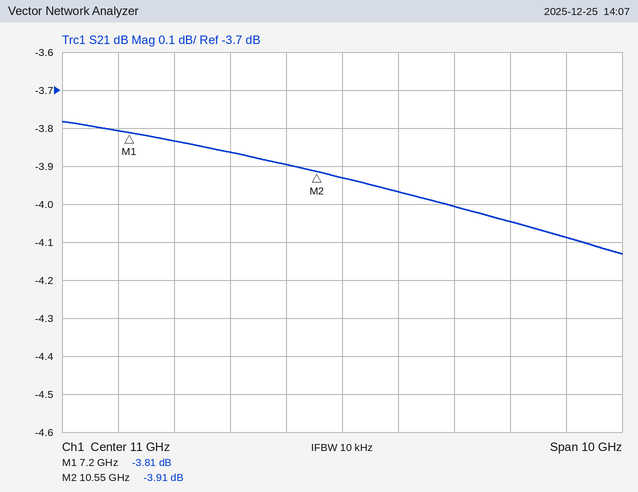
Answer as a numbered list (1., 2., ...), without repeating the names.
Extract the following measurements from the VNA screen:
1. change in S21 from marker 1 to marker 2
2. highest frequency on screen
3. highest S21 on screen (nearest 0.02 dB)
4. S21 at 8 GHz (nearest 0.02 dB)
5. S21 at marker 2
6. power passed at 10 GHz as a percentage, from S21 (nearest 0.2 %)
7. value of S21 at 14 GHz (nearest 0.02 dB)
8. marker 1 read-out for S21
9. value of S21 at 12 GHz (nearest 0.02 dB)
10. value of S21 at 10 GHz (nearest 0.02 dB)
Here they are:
1. -0.10 dB
2. 16 GHz
3. -3.78 dB
4. -3.84 dB
5. -3.91 dB
6. 40.8 %
7. -4.04 dB
8. -3.81 dB
9. -3.96 dB
10. -3.90 dB
